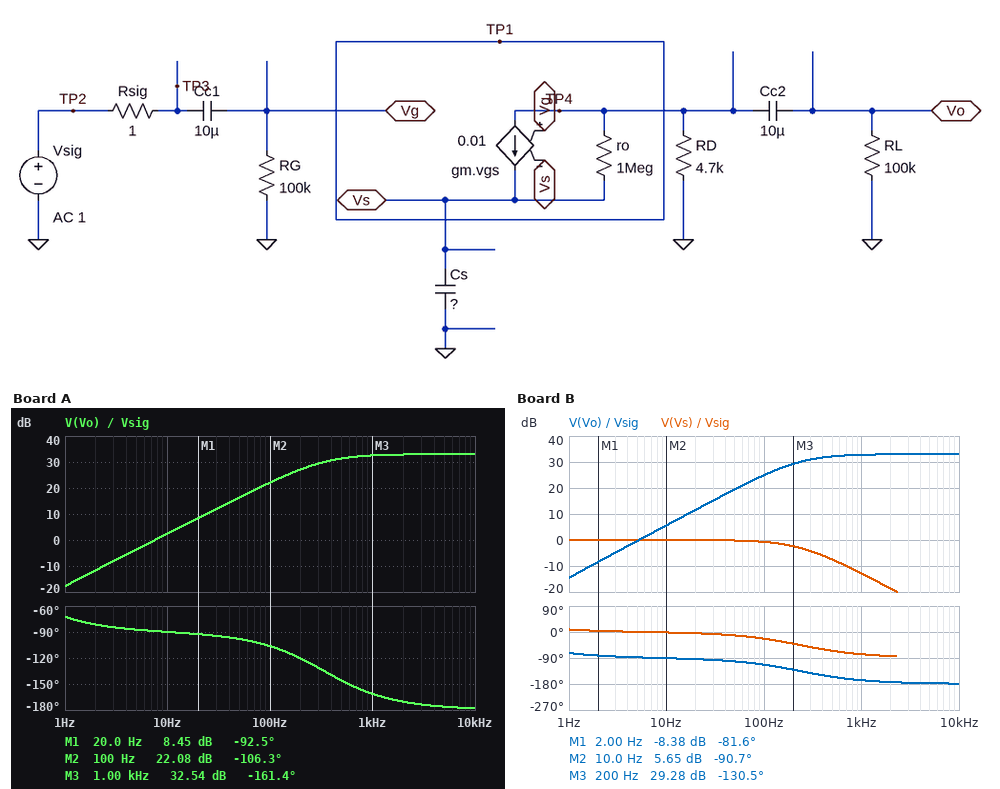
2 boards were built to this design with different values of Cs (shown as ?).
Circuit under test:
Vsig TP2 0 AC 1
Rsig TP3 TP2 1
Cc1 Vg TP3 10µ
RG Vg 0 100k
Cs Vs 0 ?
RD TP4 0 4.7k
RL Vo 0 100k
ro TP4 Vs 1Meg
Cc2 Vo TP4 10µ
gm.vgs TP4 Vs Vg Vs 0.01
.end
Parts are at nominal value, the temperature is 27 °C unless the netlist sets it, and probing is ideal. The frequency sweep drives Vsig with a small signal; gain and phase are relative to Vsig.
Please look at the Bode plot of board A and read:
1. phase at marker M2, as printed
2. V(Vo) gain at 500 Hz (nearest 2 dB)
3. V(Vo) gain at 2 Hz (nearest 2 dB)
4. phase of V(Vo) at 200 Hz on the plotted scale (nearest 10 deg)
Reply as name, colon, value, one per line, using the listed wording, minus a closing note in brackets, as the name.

phase at marker M2, as printed: -106.3 deg
V(Vo) gain at 500 Hz: 32 dB
V(Vo) gain at 2 Hz: -12 dB
phase of V(Vo) at 200 Hz on the plotted scale: -120 deg
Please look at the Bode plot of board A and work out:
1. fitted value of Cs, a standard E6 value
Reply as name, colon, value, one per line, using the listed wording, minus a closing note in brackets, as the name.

fitted value of Cs, a standard E6 value: 4.7 µF
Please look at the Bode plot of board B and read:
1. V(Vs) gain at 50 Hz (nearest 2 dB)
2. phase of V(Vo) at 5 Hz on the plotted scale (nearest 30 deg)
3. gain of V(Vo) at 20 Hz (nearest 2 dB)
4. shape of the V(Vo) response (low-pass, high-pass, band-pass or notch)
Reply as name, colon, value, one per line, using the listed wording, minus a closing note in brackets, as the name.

V(Vs) gain at 50 Hz: 0 dB
phase of V(Vo) at 5 Hz on the plotted scale: -90 deg
gain of V(Vo) at 20 Hz: 12 dB
shape of the V(Vo) response: high-pass
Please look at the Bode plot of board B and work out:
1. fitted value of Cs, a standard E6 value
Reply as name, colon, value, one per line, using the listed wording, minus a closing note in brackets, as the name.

fitted value of Cs, a standard E6 value: 6.8 µF
